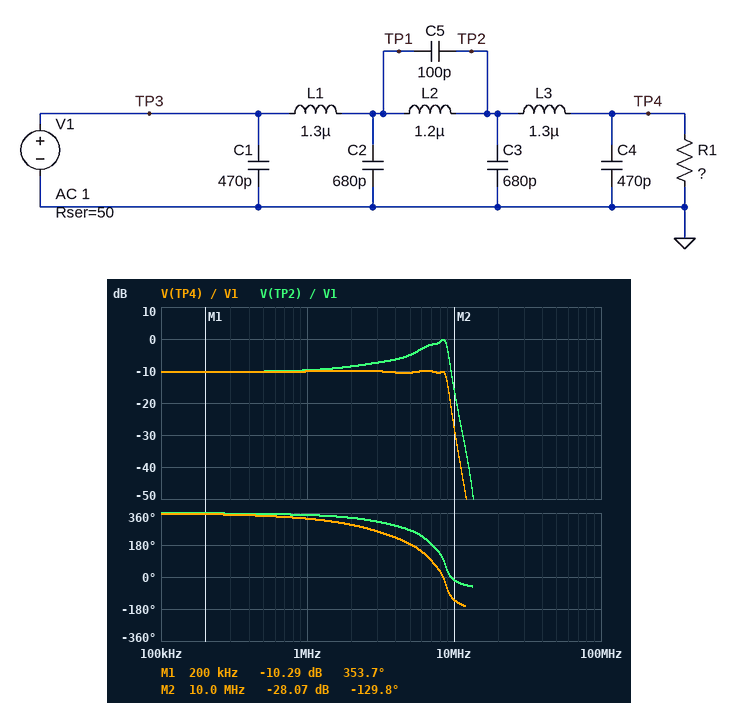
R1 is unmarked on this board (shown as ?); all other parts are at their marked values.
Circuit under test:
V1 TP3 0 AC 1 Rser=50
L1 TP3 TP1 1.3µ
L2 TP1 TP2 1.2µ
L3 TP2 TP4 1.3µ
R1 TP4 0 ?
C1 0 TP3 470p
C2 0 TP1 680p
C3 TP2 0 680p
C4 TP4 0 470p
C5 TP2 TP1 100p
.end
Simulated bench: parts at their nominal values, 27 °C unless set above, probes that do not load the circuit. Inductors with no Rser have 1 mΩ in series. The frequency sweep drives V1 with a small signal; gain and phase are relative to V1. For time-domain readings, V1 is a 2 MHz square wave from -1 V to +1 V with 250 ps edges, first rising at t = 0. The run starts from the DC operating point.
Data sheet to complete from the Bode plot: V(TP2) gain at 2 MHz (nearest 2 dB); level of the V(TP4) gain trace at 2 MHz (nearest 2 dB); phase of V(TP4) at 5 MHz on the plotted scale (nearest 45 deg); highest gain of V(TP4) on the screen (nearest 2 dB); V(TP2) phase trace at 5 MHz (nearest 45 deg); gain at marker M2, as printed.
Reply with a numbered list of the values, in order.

1. -8 dB
2. -10 dB
3. 180 deg
4. -10 dB
5. 270 deg
6. -28.07 dB
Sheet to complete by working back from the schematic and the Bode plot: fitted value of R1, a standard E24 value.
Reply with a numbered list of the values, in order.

1. 22 Ω
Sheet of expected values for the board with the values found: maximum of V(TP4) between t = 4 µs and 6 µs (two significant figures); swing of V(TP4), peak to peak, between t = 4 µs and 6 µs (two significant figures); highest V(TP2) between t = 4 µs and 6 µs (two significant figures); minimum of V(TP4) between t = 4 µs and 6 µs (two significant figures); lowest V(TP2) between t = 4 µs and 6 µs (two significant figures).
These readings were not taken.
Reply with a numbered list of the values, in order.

1. 420 mV
2. 840 mV
3. 680 mV
4. -420 mV
5. -680 mV
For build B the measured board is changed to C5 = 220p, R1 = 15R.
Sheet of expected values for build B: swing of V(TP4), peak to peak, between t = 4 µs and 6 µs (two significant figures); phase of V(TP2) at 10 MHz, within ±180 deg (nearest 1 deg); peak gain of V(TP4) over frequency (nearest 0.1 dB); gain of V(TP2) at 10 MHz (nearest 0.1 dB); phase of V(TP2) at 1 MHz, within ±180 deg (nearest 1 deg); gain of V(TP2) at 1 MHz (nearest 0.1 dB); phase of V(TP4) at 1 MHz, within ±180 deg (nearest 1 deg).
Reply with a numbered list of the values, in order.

1. 650 mV
2. 152 deg
3. -11.3 dB
4. -44.2 dB
5. -2 deg
6. -11.5 dB
7. -31 deg
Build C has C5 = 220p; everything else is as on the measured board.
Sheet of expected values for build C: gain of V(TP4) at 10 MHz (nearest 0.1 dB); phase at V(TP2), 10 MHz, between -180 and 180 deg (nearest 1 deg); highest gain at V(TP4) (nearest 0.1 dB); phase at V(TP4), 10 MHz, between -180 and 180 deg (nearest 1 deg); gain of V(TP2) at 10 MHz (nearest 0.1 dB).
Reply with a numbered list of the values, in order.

1. -56.1 dB
2. 154 deg
3. -9.6 dB
4. 43 deg
5. -44.1 dB
